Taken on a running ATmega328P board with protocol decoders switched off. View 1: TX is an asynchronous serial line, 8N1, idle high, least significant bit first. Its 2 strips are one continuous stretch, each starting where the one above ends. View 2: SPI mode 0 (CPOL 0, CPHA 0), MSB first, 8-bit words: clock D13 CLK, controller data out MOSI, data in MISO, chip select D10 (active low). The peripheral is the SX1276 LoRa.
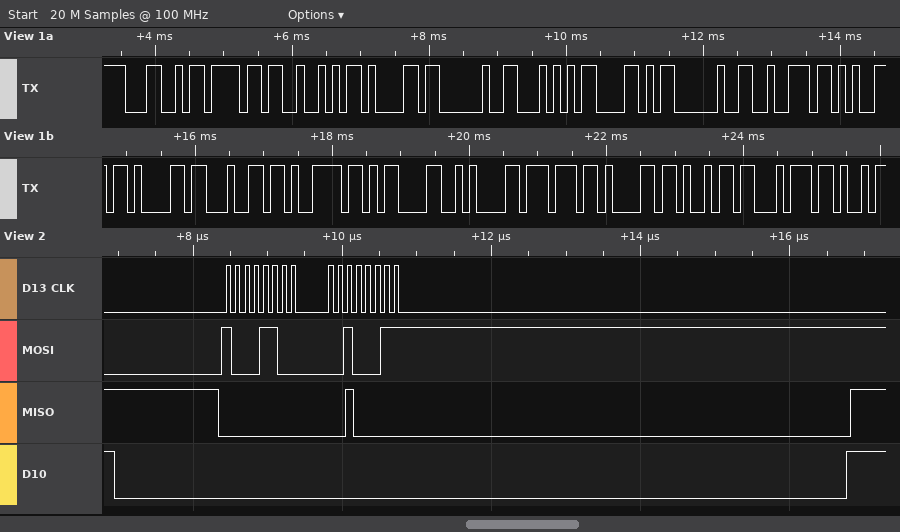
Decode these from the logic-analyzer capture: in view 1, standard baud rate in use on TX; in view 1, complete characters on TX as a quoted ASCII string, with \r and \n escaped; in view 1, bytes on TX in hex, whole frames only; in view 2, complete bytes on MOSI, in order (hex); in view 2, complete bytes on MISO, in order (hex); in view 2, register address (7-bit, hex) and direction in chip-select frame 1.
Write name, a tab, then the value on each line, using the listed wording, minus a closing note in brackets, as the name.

in view 1, standard baud rate in use on TX	9600 baud
in view 1, complete characters on TX as a quoted ASCII string, with \r and \n escaped	"LoRa TX ready\r\nwait"
in view 1, bytes on TX in hex, whole frames only	4C 6F 52 61 20 54 58 20 72 65 61 64 79 0D 0A 77 61 69 74
in view 2, complete bytes on MOSI, in order	8C 23
in view 2, complete bytes on MISO, in order	00 20
in view 2, register address (7-bit, hex) and direction in chip-select frame 1	0x0C write
